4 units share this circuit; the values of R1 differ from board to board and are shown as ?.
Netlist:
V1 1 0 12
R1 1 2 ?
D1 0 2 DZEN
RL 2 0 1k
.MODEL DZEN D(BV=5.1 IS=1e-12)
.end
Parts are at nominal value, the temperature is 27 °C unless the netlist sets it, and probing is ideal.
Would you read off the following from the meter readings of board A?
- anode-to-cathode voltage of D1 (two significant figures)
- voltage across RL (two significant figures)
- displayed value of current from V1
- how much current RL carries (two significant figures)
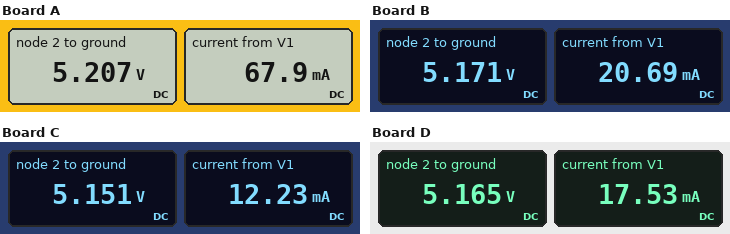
-5.2 V
5.2 V
67.9 mA
5.2 mA
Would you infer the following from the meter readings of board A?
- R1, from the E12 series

100 Ω
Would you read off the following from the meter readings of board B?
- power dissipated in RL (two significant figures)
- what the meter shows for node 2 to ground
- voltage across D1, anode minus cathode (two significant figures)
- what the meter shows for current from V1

27 mW
5.171 V
-5.2 V
20.69 mA
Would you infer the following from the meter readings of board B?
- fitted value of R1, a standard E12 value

330 Ω
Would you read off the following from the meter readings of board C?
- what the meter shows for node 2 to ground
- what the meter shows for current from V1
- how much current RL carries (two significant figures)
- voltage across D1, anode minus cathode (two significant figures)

5.151 V
12.23 mA
5.2 mA
-5.2 V
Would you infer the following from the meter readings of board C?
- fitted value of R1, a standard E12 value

560 Ω
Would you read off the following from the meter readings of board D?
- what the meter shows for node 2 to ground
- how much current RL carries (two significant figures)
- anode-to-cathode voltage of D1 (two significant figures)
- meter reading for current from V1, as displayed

5.165 V
5.2 mA
-5.2 V
17.53 mA
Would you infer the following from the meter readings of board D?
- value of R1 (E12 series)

390 Ω
